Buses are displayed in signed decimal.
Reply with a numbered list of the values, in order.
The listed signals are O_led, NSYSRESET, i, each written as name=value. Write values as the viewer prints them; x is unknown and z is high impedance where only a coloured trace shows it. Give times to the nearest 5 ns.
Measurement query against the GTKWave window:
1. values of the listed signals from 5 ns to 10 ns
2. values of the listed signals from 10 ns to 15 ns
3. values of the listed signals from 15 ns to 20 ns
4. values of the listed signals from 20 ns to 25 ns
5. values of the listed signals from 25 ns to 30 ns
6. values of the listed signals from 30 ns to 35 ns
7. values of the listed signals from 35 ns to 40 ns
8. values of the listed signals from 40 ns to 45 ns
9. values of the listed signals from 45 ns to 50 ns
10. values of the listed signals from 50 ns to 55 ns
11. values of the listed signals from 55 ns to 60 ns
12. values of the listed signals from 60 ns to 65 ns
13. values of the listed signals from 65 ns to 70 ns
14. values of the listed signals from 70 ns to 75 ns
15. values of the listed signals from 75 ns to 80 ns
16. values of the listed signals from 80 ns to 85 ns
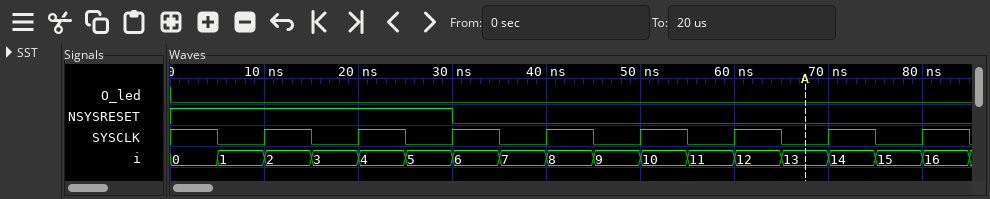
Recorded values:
1. O_led=0, NSYSRESET=1, i=1
2. O_led=0, NSYSRESET=1, i=2
3. O_led=0, NSYSRESET=1, i=3
4. O_led=0, NSYSRESET=1, i=4
5. O_led=0, NSYSRESET=1, i=5
6. O_led=0, NSYSRESET=0, i=6
7. O_led=0, NSYSRESET=0, i=7
8. O_led=0, NSYSRESET=0, i=8
9. O_led=0, NSYSRESET=0, i=9
10. O_led=0, NSYSRESET=0, i=10
11. O_led=0, NSYSRESET=0, i=11
12. O_led=0, NSYSRESET=0, i=12
13. O_led=0, NSYSRESET=0, i=13
14. O_led=0, NSYSRESET=0, i=14
15. O_led=0, NSYSRESET=0, i=15
16. O_led=0, NSYSRESET=0, i=16
